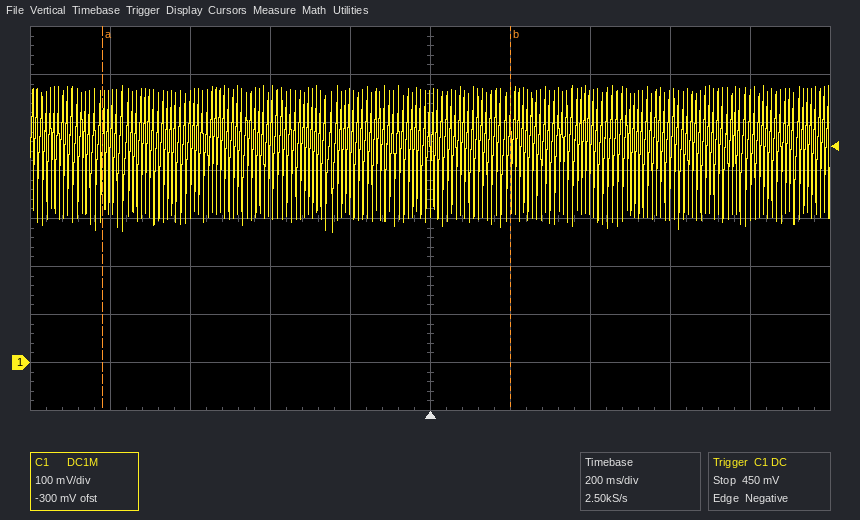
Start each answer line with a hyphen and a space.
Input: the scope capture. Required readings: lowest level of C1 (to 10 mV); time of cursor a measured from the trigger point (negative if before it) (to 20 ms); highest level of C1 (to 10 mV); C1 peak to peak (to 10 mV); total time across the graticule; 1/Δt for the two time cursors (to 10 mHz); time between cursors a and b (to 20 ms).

- 270 mV
- -820 ms
- 580 mV
- 310 mV
- 2 s
- 980 mHz
- 1.02 s
